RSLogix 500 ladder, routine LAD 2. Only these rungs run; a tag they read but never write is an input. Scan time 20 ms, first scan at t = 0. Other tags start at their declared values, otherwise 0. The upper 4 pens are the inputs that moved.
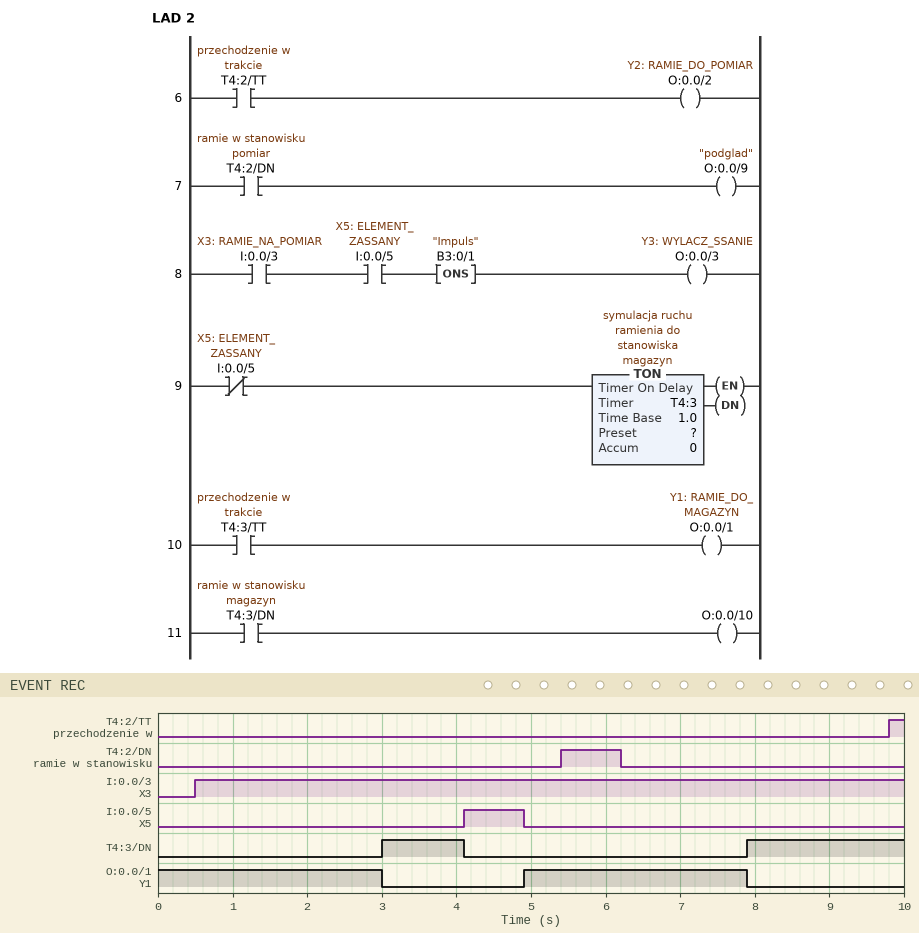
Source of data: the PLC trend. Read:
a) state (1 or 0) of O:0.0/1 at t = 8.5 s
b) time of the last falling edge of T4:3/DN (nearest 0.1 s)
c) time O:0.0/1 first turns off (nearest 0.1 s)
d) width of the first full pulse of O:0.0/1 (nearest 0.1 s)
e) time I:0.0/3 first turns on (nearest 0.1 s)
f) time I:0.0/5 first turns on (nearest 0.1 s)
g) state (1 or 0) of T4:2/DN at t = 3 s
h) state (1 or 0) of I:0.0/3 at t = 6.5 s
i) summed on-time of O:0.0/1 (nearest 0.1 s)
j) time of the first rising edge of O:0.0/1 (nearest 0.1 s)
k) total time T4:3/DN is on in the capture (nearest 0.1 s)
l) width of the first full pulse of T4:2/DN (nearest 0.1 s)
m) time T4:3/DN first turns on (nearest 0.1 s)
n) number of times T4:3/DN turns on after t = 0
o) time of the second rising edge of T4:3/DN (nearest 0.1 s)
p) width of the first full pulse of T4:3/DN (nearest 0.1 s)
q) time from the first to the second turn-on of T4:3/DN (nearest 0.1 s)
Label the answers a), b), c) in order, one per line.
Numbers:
a) 0
b) 4.1 s
c) 3.0 s
d) 3.0 s
e) 0.5 s
f) 4.1 s
g) 0
h) 1
i) 6.0 s
j) 4.9 s
k) 3.2 s
l) 0.8 s
m) 3.0 s
n) 2
o) 7.9 s
p) 1.1 s
q) 4.9 s
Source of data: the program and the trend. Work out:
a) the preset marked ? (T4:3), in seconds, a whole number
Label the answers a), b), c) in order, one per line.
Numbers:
a) 3 s
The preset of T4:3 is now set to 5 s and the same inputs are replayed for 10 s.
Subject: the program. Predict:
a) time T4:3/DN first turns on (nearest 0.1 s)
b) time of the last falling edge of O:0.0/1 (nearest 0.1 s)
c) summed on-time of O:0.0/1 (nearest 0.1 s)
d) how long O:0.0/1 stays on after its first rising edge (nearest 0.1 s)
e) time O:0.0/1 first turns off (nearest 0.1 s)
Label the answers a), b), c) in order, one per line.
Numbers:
a) 9.9 s
b) 9.9 s
c) 9.1 s
d) 5.0 s
e) 4.1 s
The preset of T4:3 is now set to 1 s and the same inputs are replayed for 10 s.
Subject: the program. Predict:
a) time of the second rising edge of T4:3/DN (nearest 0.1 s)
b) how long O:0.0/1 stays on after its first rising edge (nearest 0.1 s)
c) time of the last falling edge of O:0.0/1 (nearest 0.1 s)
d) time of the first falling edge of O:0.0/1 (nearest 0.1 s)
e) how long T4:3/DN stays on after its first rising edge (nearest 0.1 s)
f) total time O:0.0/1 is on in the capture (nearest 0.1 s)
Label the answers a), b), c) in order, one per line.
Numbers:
a) 5.9 s
b) 1.0 s
c) 5.9 s
d) 1.0 s
e) 3.1 s
f) 2.0 s
